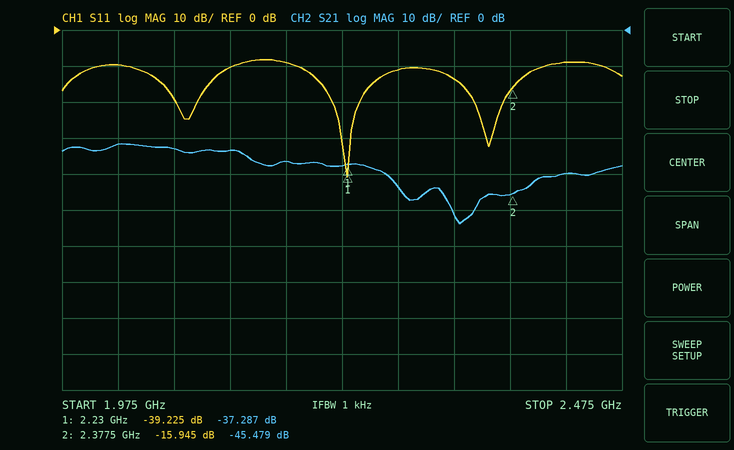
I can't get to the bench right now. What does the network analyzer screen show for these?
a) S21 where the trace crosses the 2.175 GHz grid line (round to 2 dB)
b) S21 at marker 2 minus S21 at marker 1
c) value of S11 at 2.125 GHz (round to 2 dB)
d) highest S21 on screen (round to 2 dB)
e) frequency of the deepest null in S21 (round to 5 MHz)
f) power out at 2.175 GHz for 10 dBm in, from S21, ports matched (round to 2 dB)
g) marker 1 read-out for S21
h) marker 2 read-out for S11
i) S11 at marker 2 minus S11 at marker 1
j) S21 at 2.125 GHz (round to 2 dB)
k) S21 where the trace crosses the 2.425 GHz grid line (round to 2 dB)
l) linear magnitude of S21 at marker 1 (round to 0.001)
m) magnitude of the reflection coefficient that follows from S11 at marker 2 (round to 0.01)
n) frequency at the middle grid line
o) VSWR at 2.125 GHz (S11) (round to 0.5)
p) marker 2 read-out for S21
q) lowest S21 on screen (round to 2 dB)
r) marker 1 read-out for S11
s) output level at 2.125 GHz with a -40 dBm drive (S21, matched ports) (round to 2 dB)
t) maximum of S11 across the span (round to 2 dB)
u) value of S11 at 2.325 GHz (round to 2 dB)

-36 dB
-8.192 dB
-10 dB
-32 dB
2.330 GHz
-26 dBm
-37.287 dB
-15.945 dB
23.280 dB
-34 dB
-40 dB
0.014
0.16
2.225 GHz
2.0
-45.479 dB
-54 dB
-39.225 dB
-74 dBm
-8 dB
-14 dB
